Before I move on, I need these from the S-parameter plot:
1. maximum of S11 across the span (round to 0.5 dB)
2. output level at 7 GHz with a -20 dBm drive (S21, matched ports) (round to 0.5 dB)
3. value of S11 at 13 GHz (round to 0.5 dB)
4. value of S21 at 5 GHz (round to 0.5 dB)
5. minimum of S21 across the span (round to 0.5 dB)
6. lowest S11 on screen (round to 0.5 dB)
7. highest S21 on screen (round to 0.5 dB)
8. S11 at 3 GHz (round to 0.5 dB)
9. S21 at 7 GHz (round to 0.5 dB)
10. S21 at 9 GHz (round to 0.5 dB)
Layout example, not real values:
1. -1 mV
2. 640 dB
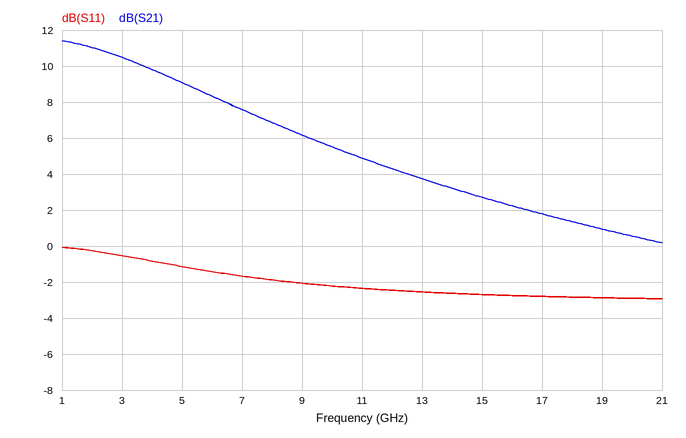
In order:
1. 0.0 dB
2. -12.5 dBm
3. -2.5 dB
4. 9.0 dB
5. 0.0 dB
6. -3.0 dB
7. 11.5 dB
8. -0.5 dB
9. 7.5 dB
10. 6.0 dB
